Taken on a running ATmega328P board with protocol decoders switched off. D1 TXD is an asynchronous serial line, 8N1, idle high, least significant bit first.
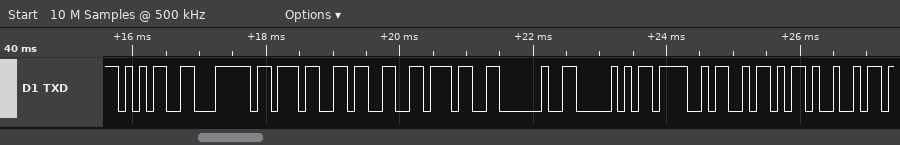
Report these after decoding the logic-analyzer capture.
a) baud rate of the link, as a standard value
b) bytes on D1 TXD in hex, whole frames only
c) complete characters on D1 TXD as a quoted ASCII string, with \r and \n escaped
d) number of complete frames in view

9600 baud
35 7C 37 33 37 20 50 4F 5A 49
"5|737 POZI"
10
